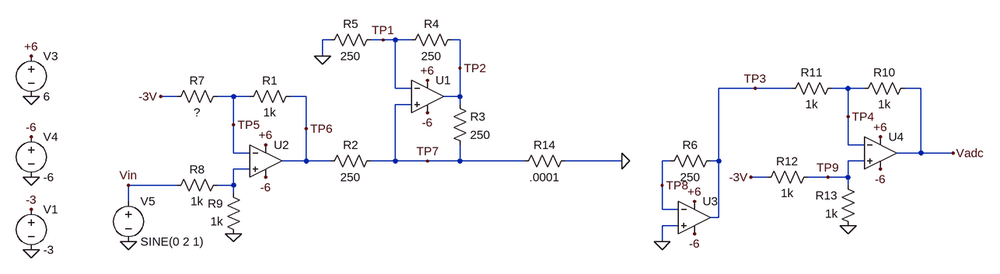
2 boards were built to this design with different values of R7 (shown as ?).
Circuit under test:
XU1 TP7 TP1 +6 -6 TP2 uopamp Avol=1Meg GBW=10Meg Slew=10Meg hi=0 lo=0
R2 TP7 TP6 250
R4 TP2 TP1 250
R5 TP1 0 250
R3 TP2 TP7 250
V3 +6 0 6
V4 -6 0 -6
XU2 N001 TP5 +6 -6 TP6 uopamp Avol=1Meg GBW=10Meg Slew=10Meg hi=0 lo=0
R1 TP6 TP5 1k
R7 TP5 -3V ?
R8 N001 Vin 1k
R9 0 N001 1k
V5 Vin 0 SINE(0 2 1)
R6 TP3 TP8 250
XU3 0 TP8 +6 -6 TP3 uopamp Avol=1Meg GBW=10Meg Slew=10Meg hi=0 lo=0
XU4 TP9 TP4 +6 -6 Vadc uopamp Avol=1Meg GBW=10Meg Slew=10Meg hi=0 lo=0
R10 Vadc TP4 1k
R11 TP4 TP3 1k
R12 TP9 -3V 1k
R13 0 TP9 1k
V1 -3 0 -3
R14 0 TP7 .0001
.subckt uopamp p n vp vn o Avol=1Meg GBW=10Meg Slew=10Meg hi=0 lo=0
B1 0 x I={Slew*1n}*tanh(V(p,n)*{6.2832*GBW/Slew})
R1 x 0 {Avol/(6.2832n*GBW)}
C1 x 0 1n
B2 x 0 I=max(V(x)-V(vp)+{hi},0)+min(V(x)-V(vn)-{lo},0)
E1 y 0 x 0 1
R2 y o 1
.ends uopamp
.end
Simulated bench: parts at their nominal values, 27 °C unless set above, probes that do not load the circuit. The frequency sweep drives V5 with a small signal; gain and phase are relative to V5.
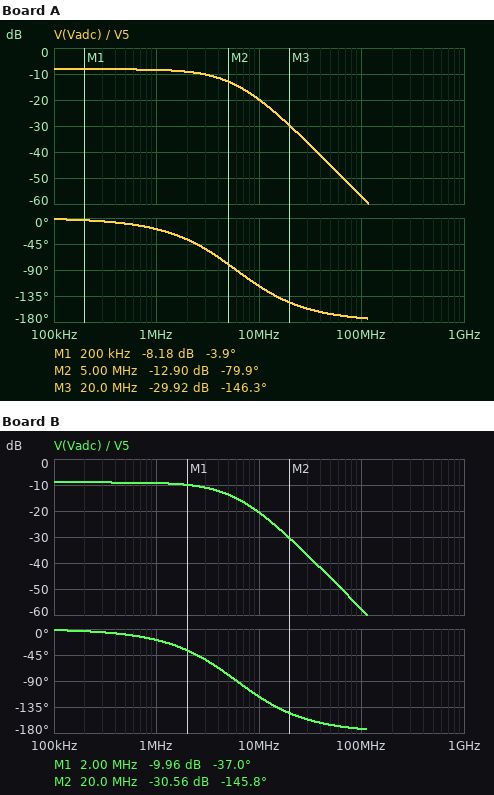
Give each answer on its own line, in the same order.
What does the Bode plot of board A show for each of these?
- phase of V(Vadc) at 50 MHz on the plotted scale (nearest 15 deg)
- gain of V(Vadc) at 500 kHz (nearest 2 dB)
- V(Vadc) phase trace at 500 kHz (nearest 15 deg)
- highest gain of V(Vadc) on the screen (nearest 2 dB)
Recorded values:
-165 deg
-8 dB
-15 deg
-8 dB
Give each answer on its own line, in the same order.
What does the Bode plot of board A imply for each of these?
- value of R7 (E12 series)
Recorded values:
560 Ω
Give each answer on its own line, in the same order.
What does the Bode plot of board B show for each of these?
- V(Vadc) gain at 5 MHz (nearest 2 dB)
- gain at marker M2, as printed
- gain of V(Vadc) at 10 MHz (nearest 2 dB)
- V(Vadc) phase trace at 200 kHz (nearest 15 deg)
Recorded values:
-14 dB
-30.56 dB
-20 dB
0 deg
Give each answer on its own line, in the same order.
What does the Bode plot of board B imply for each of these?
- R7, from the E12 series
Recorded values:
820 Ω
